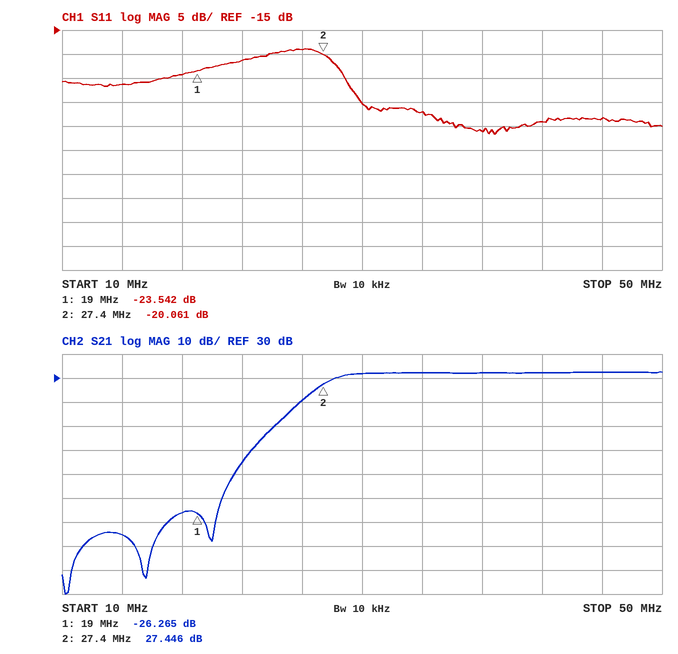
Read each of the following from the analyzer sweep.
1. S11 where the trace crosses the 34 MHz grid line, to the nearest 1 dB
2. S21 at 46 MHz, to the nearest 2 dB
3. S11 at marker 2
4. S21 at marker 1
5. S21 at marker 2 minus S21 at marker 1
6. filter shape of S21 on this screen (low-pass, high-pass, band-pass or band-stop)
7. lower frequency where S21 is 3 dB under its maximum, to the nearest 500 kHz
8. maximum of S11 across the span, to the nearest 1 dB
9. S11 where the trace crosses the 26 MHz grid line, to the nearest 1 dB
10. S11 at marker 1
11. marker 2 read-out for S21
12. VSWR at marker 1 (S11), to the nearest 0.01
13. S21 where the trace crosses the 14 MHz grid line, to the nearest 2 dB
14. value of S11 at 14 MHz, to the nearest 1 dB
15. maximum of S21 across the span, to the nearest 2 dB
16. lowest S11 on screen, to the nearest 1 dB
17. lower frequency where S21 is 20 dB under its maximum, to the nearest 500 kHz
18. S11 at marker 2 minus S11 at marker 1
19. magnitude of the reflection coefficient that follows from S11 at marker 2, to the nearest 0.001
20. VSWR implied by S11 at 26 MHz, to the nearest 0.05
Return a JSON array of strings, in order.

["-32 dB", "32 dB", "-20.061 dB", "-26.265 dB", "53.711 dB", "high-pass", "28.0 MHz", "-19 dB", "-19 dB", "-23.542 dB", "27.446 dB", "1.14", "-36 dB", "-26 dB", "32 dB", "-37 dB", "24.5 MHz", "3.481 dB", "0.099", "1.25"]
